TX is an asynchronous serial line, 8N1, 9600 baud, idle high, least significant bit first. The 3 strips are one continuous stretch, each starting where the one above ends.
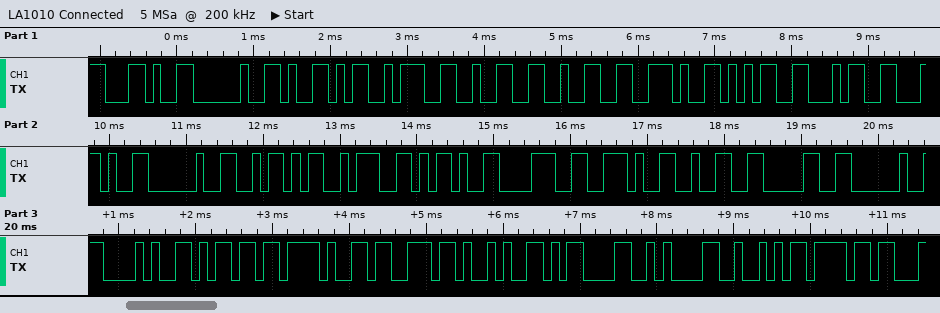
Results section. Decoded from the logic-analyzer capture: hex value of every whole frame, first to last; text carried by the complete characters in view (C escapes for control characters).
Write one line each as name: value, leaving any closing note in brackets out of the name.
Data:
hex value of every whole frame, first to last: 0x2C 0x20 0x59 0x3A 0x32 0x32 0x2E 0x35 0x34 0x2C 0x20 0x5A 0x3A 0x2D 0x38 0x2E 0x32 0x30 0x20 0x28 0x6D 0x2F 0x73 0x29 0x0D 0x0A 0x52 0x6F
text carried by the complete characters in view: ", Y:22.54, Z:-8.20 (m/s)\r\nRo"
